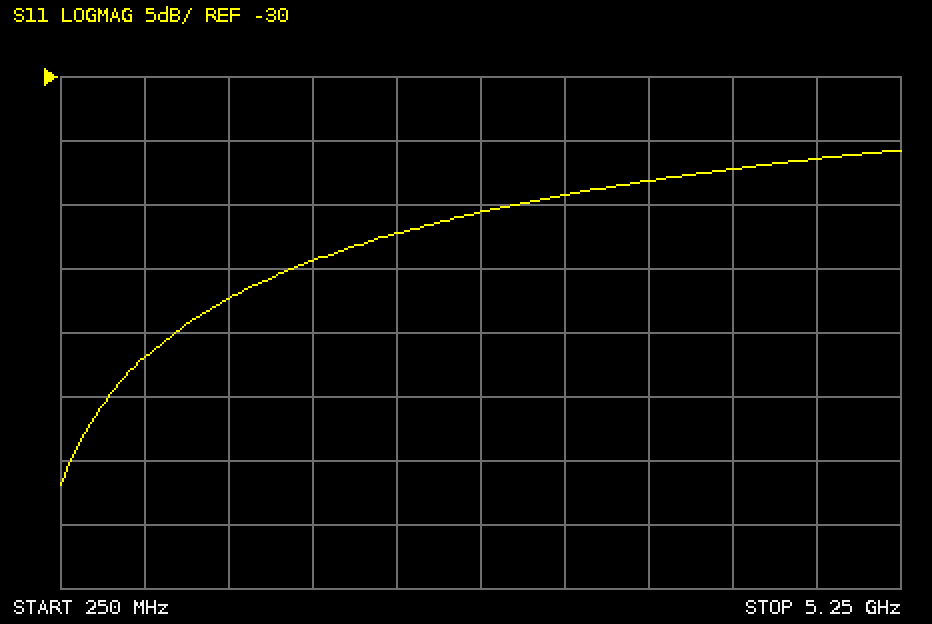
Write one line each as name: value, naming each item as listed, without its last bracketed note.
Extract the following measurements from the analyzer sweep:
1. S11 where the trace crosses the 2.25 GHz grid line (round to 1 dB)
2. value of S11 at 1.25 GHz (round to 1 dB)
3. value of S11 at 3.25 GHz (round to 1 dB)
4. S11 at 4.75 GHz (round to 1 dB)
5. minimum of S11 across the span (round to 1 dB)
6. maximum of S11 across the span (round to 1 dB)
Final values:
S11 where the trace crosses the 2.25 GHz grid line: -42 dB
value of S11 at 1.25 GHz: -47 dB
value of S11 at 3.25 GHz: -39 dB
S11 at 4.75 GHz: -36 dB
minimum of S11 across the span: -62 dB
maximum of S11 across the span: -36 dB
